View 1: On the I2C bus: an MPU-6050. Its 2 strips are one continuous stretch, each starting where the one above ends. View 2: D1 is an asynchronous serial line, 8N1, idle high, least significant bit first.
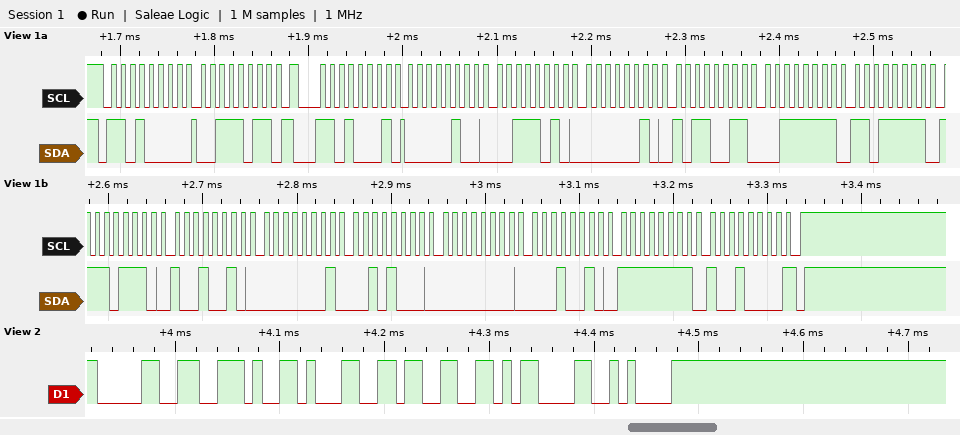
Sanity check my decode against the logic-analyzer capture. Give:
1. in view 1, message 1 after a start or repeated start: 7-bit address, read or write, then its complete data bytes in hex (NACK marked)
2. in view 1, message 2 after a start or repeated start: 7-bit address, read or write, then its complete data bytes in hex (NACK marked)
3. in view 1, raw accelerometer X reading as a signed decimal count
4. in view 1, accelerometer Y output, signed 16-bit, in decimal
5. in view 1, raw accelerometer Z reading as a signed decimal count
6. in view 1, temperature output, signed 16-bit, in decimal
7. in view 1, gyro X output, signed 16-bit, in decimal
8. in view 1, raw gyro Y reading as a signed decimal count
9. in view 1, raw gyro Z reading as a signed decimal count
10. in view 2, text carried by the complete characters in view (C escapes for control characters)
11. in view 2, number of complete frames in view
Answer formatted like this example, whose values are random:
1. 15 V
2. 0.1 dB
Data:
1. 0x68 write: 3B
2. 0x68 read: 04 3A 02 B3 3F DF EE 92 01 28 00 12 FF 90 NACK
3. 1082
4. 691
5. 16351
6. -4462
7. 296
8. 18
9. -112
10. "0.13\r\n"
11. 6
